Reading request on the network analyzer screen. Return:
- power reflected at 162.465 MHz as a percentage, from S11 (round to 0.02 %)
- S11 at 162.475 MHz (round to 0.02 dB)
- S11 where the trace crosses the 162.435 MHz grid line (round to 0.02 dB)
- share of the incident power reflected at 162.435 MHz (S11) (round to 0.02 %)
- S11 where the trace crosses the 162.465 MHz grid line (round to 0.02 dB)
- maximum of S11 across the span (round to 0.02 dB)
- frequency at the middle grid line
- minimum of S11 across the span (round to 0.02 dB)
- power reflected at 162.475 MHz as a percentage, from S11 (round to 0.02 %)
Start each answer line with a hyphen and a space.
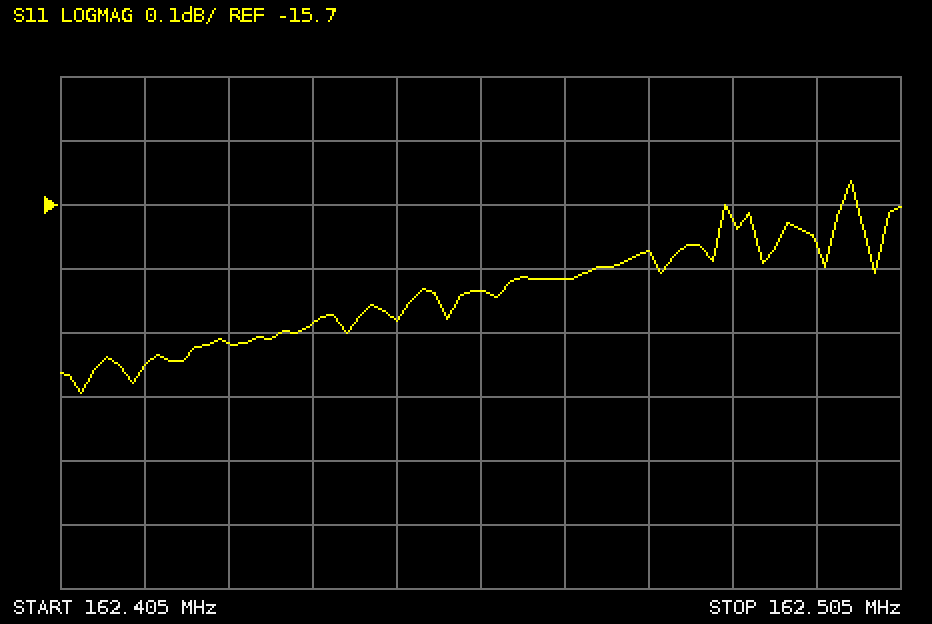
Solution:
- 2.62 %
- -15.78 dB
- -15.88 dB
- 2.58 %
- -15.82 dB
- -15.66 dB
- 162.455 MHz
- -16.00 dB
- 2.64 %
